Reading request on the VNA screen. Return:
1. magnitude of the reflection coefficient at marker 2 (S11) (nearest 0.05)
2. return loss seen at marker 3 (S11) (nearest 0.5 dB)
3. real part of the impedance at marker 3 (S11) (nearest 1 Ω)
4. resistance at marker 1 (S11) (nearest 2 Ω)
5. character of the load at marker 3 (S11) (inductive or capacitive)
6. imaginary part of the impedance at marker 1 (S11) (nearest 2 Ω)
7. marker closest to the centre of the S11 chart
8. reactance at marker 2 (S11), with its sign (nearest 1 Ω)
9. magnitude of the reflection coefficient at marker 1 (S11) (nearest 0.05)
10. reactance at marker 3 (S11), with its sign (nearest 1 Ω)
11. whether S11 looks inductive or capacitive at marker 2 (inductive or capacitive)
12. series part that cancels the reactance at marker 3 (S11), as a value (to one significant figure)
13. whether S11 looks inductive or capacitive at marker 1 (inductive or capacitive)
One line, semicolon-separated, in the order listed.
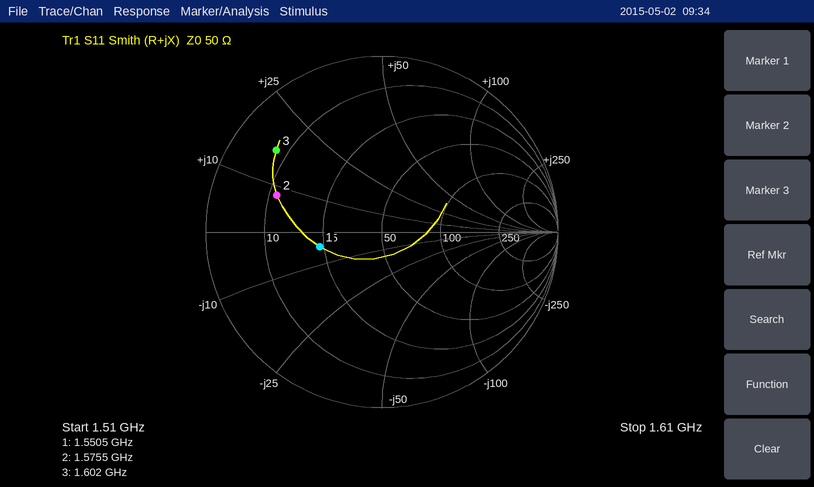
0.65; 2.5 dB; 8 Ω; 24 Ω; inductive; -4 Ω; marker 1; +8 Ω; 0.35; +17 Ω; inductive; 6 pF; capacitive
